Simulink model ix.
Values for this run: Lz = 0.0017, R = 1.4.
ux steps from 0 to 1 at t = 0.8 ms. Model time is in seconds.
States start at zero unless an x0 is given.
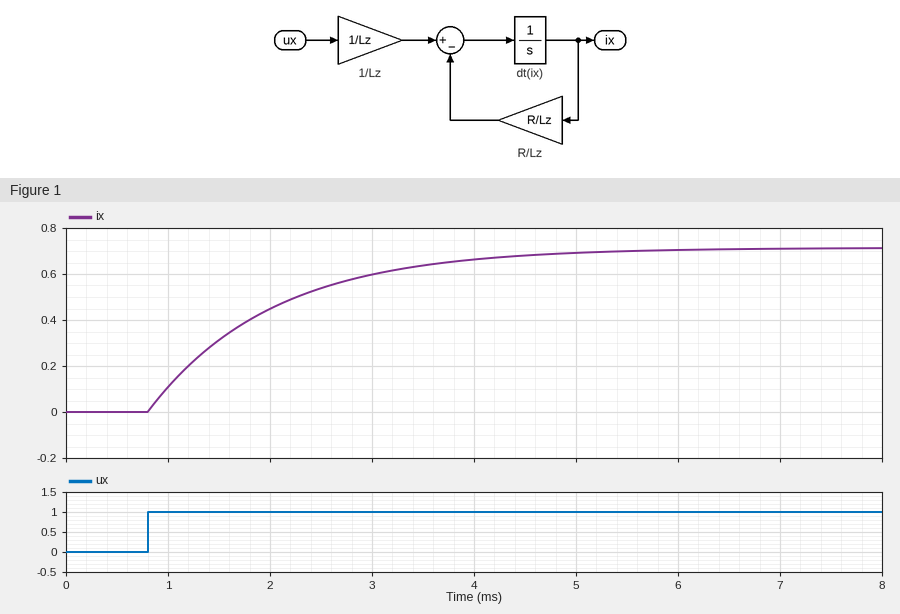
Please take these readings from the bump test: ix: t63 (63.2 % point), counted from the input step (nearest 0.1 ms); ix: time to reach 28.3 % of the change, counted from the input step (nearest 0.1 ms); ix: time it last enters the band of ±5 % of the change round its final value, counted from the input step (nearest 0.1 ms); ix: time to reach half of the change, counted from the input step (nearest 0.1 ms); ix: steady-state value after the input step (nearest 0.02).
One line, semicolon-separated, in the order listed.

1.2 ms; 0.4 ms; 3.6 ms; 0.8 ms; 0.72
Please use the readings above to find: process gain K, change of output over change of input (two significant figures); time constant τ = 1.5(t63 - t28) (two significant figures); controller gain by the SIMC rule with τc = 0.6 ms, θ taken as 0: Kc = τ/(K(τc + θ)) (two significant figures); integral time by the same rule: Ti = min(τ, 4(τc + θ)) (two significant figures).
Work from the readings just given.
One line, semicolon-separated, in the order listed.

0.72; 1.2 ms; 2.8; 1.2 ms
